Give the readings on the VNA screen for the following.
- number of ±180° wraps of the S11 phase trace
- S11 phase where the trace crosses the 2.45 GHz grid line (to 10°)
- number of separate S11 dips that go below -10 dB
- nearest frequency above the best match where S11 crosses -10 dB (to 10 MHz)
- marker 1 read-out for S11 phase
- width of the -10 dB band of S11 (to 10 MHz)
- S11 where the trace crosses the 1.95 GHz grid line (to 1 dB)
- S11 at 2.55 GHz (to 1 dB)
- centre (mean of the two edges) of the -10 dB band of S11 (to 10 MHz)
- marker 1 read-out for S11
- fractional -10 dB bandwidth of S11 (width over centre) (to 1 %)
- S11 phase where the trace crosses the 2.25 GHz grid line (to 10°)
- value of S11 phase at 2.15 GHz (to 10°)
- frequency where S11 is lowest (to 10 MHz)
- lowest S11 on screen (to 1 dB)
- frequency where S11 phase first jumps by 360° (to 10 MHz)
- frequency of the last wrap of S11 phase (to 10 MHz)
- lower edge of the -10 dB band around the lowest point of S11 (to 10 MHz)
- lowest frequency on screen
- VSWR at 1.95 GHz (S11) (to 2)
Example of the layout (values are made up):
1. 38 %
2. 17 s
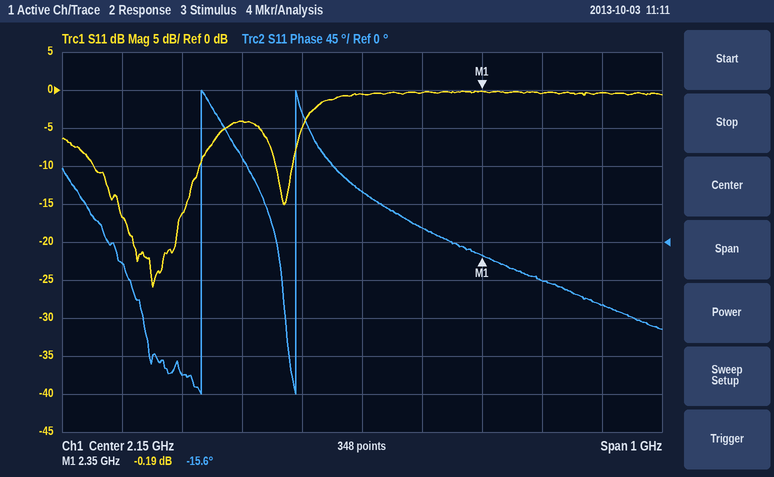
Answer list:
1. 2
2. -50°
3. 2
4. 1.88 GHz
5. -15.6°
6. 180 MHz
7. -4 dB
8. 0 dB
9. 1.79 GHz
10. -0.19 dB
11. 10 %
12. 20°
13. 60°
14. 1.80 GHz
15. -26 dB
16. 1.88 GHz
17. 2.04 GHz
18. 1.70 GHz
19. 1.65 GHz
20. 4
